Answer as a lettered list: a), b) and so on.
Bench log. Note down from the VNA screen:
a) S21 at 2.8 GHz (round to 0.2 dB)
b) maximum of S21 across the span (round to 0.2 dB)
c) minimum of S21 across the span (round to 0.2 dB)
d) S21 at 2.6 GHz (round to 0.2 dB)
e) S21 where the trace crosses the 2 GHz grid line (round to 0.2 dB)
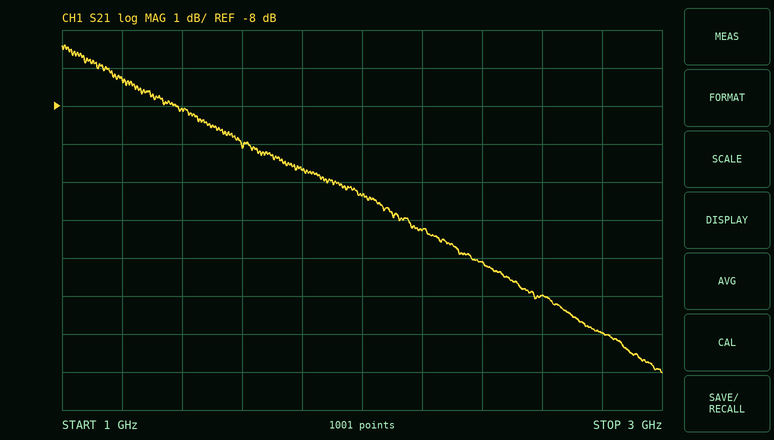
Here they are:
a) -14.0 dB
b) -6.4 dB
c) -15.0 dB
d) -13.0 dB
e) -10.4 dB
